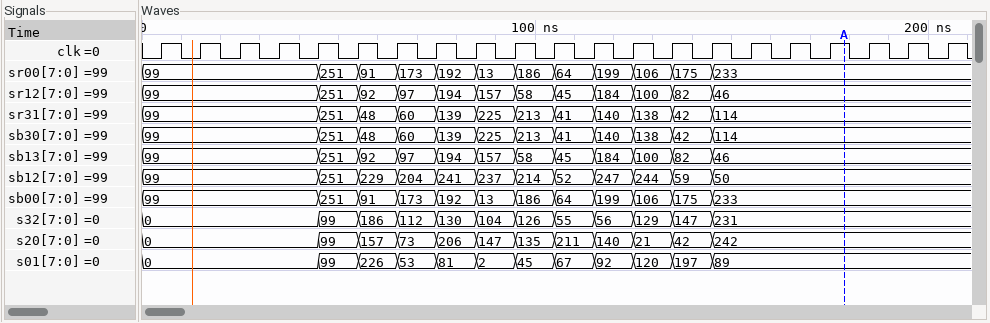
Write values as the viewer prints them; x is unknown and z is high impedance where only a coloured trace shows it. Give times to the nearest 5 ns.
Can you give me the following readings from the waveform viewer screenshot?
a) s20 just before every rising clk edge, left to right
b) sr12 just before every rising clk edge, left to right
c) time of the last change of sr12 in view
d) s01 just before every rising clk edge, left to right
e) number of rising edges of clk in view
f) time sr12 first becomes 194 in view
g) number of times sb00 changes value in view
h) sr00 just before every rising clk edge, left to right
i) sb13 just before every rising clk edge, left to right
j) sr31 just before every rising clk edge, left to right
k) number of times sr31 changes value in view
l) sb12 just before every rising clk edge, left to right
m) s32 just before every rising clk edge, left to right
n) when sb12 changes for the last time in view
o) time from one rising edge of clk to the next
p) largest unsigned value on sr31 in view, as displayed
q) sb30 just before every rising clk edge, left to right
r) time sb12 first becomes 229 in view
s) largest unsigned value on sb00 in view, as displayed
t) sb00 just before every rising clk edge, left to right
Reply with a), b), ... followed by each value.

a) 0, 0, 0, 0, 0, 99, 157, 73, 206, 147, 135, 211, 140, 21, 42, 242, 242, 242, 242, 242, 242
b) 99, 99, 99, 99, 99, 251, 92, 97, 194, 157, 58, 45, 184, 100, 82, 46, 46, 46, 46, 46, 46
c) 145 ns
d) 0, 0, 0, 0, 0, 99, 226, 53, 81, 2, 45, 67, 92, 120, 197, 89, 89, 89, 89, 89, 89
e) 21
f) 75 ns
g) 11
h) 99, 99, 99, 99, 99, 251, 91, 173, 192, 13, 186, 64, 199, 106, 175, 233, 233, 233, 233, 233, 233
i) 99, 99, 99, 99, 99, 251, 92, 97, 194, 157, 58, 45, 184, 100, 82, 46, 46, 46, 46, 46, 46
j) 99, 99, 99, 99, 99, 251, 48, 60, 139, 225, 213, 41, 140, 138, 42, 114, 114, 114, 114, 114, 114
k) 11
l) 99, 99, 99, 99, 99, 251, 229, 204, 241, 237, 214, 52, 247, 244, 59, 50, 50, 50, 50, 50, 50
m) 0, 0, 0, 0, 0, 99, 186, 112, 130, 104, 126, 55, 56, 129, 147, 231, 231, 231, 231, 231, 231
n) 145 ns
o) 10 ns
p) 251
q) 99, 99, 99, 99, 99, 251, 48, 60, 139, 225, 213, 41, 140, 138, 42, 114, 114, 114, 114, 114, 114
r) 55 ns
s) 251
t) 99, 99, 99, 99, 99, 251, 91, 173, 192, 13, 186, 64, 199, 106, 175, 233, 233, 233, 233, 233, 233
